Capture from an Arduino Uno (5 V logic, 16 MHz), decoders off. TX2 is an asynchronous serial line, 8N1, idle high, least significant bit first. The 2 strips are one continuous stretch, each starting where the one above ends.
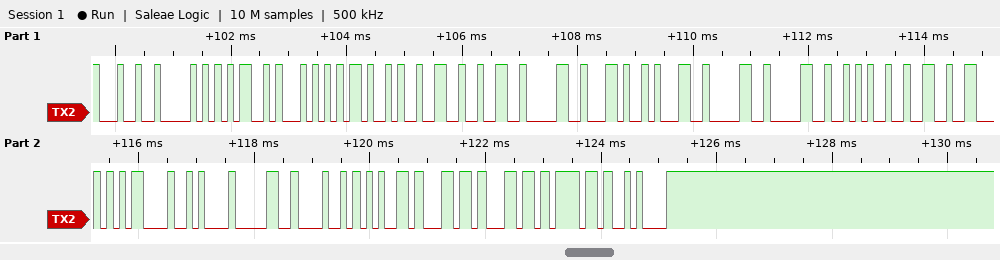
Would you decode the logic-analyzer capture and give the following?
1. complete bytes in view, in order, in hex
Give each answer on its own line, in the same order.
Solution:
0x24 0x50 0x4D 0x54 0x4B 0x32 0x32 0x30 0x2C 0x31 0x30 0x30 0x2A 0x32 0x46 0x0D 0x0A 0x30 0x48 0x65 0x6C 0x6C 0x6F 0x0A
